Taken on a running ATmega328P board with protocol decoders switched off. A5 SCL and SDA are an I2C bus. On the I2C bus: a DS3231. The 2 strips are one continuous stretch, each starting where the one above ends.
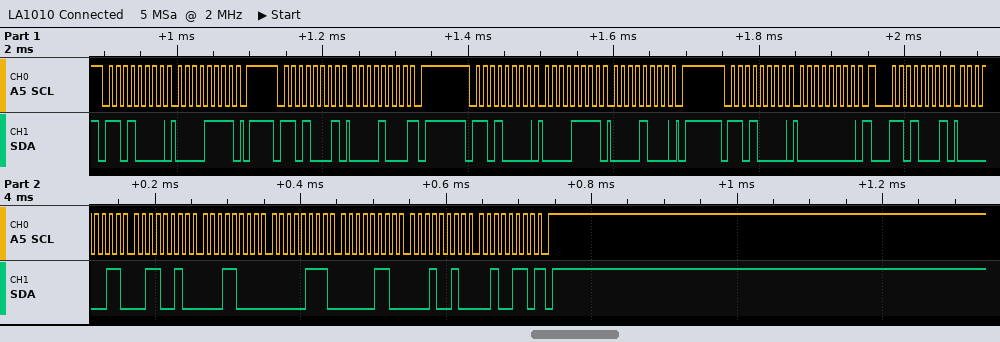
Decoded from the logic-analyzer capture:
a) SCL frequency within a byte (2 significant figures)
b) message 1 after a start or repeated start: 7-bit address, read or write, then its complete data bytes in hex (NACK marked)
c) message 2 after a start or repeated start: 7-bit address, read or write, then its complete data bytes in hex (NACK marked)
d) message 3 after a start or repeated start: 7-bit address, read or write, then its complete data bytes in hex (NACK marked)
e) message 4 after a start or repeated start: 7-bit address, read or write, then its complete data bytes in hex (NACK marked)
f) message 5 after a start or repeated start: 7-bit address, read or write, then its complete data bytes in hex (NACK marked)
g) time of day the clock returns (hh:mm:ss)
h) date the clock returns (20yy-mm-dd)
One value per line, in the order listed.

100 kHz
0x68 write: 0F
0x68 read: 08 NACK
0x68 write: 0F 08
0x68 write: 00
0x68 read: 03 32 18 07 06 12 26 NACK
18:32:03
2026-12-06
